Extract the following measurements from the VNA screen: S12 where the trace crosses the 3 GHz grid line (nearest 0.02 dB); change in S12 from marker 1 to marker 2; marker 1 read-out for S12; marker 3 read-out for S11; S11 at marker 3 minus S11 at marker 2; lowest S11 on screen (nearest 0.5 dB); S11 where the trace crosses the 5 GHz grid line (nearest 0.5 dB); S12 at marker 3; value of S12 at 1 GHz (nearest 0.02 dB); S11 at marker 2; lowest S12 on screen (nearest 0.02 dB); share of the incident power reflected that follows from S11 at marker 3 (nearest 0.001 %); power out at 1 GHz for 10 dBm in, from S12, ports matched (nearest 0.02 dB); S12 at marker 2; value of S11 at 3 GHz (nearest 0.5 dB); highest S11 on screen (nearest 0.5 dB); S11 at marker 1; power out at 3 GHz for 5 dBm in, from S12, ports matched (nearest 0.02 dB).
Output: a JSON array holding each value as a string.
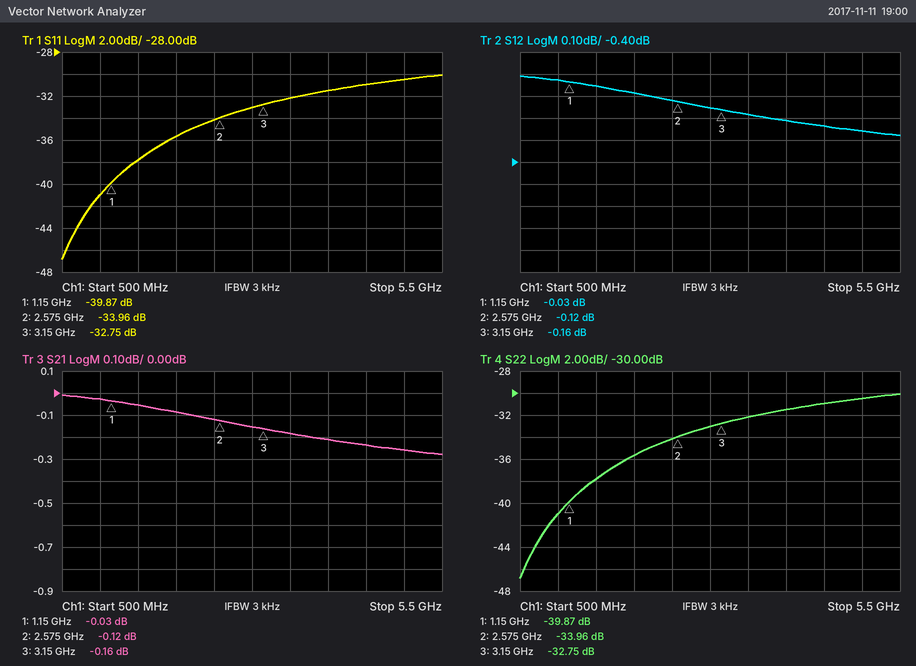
["-0.16 dB", "-0.09 dB", "-0.03 dB", "-32.75 dB", "1.21 dB", "-47.0 dB", "-30.5 dB", "-0.16 dB", "-0.02 dB", "-33.96 dB", "-0.28 dB", "0.053 %", "9.98 dBm", "-0.12 dB", "-33.0 dB", "-30.0 dB", "-39.87 dB", "4.84 dBm"]
